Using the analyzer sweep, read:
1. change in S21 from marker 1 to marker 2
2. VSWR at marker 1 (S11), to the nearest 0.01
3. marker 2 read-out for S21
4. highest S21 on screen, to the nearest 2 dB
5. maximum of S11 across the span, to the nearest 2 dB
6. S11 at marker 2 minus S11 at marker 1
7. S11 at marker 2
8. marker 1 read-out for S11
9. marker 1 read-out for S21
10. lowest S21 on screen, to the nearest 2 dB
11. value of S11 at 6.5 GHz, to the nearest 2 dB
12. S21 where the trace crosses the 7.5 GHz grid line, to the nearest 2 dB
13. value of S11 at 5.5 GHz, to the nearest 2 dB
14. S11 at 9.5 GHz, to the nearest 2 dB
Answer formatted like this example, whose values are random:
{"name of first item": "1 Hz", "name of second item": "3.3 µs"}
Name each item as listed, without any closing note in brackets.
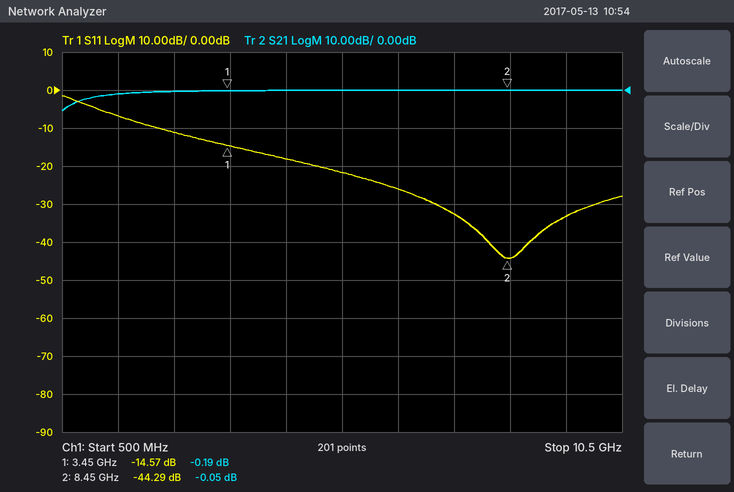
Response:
{"change in S21 from marker 1 to marker 2": "0.14 dB", "VSWR at marker 1 (S11), to the nearest 0.01": "1.46", "marker 2 read-out for S21": "-0.05 dB", "highest S21 on screen, to the nearest 2 dB": "0 dB", "maximum of S11 across the span, to the nearest 2 dB": "-2 dB", "S11 at marker 2 minus S11 at marker 1": "-29.72 dB", "S11 at marker 2": "-44.29 dB", "marker 1 read-out for S11": "-14.57 dB", "marker 1 read-out for S21": "-0.19 dB", "lowest S21 on screen, to the nearest 2 dB": "-6 dB", "value of S11 at 6.5 GHz, to the nearest 2 dB": "-26 dB", "S21 where the trace crosses the 7.5 GHz grid line, to the nearest 2 dB": "0 dB", "value of S11 at 5.5 GHz, to the nearest 2 dB": "-22 dB", "S11 at 9.5 GHz, to the nearest 2 dB": "-34 dB"}
